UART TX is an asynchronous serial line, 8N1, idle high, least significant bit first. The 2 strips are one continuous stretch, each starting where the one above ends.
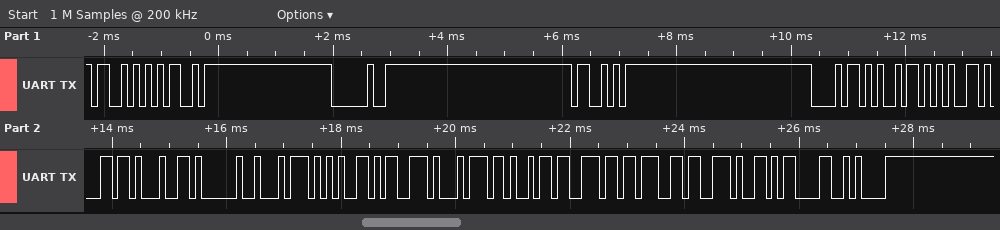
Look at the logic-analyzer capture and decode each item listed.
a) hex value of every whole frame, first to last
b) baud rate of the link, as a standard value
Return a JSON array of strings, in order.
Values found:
["0x53 0x4D 0x20 0x53 0x68 0x69 0x65 0x6C 0x64 0x20 0x74 0x65 0x73 0x74 0x69 0x6E 0x67 0x2E 0x0D 0x0A", "9600 baud"]
